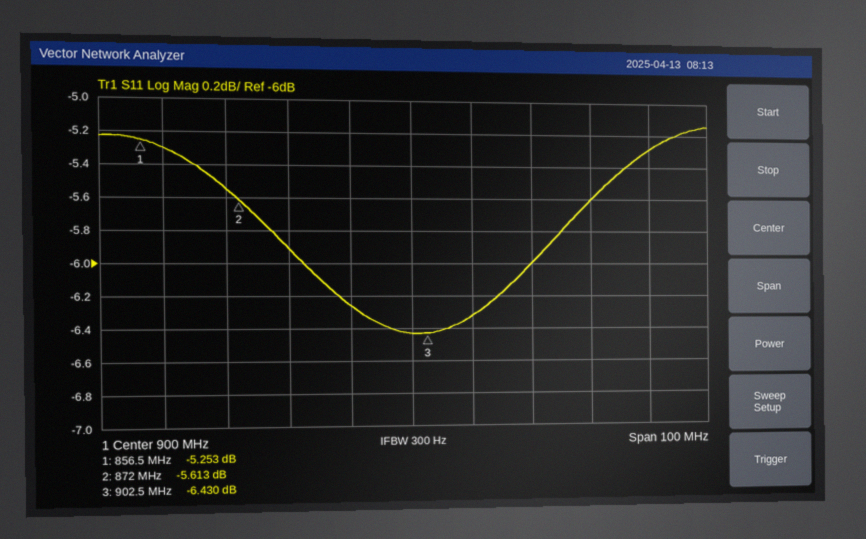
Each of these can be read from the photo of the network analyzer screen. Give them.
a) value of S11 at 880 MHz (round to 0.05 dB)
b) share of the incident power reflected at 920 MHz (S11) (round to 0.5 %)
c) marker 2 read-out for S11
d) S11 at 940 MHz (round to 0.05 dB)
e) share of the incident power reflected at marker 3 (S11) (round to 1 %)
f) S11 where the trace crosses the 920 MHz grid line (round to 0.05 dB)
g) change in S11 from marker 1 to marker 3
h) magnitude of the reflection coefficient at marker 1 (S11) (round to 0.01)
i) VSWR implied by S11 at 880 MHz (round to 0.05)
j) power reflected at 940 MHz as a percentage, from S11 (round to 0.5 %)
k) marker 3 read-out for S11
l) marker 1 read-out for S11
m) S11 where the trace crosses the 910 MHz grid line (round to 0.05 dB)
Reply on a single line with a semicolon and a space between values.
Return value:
-5.90 dB; 25.0 %; -5.613 dB; -5.30 dB; 23 %; -6.00 dB; -1.177 dB; 0.55; 3.05; 29.5 %; -6.430 dB; -5.253 dB; -6.30 dB
